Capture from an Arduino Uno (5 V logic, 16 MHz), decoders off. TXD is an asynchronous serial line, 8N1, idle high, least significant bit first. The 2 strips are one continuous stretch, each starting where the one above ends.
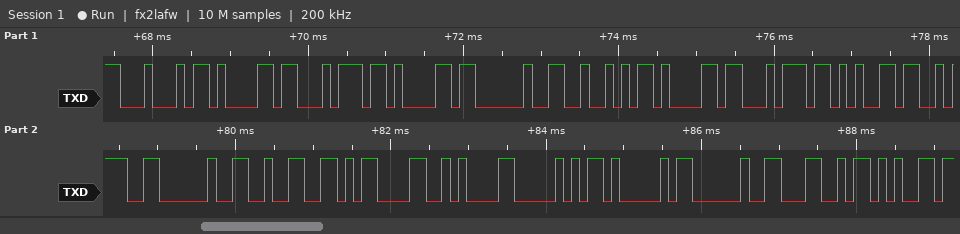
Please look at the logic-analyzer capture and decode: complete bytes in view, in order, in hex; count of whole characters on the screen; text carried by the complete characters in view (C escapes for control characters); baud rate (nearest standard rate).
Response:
0x44 0x61 0x74 0x61 0x20 0x52 0x61 0x74 0x65 0x3A 0x20 0x32 0x0D 0x0A 0x50 0x41 0x20 0x4C 0x65
19
"Data Rate: 2\r\nPA Le"
9600 baud
